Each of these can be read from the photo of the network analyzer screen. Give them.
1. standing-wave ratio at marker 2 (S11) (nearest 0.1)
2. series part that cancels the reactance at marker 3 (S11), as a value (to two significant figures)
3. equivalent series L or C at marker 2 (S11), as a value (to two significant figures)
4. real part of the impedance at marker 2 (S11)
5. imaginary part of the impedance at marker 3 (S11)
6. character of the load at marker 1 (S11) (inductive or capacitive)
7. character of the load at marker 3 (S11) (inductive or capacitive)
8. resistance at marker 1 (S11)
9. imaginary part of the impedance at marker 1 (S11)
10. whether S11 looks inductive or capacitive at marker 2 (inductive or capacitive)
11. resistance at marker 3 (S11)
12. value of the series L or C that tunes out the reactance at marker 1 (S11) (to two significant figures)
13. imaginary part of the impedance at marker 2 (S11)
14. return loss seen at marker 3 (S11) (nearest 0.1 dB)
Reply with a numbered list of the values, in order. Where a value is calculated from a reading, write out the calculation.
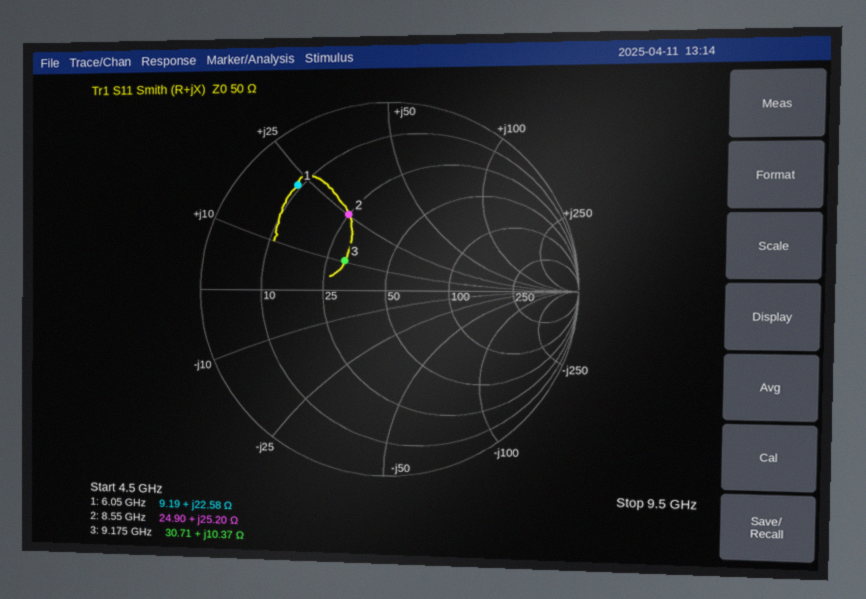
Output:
1. 2.6
2. C = 1/(2π × 9.175 GHz × 10.37 Ω) ≈ 1.7 pF
3. L = 25.2 Ω/(2π × 8.55 GHz) ≈ 469 pH, so 470 pH to two significant figures
4. 24.90 Ω
5. +10.37 Ω
6. inductive
7. inductive
8. 9.19 Ω
9. +22.58 Ω
10. inductive
11. 30.71 Ω
12. C = 1/(2π × 6.05 GHz × 22.58 Ω) ≈ 1.2 pF
13. +25.20 Ω
14. 11.4 dB
